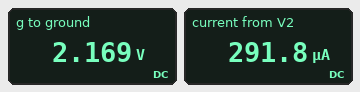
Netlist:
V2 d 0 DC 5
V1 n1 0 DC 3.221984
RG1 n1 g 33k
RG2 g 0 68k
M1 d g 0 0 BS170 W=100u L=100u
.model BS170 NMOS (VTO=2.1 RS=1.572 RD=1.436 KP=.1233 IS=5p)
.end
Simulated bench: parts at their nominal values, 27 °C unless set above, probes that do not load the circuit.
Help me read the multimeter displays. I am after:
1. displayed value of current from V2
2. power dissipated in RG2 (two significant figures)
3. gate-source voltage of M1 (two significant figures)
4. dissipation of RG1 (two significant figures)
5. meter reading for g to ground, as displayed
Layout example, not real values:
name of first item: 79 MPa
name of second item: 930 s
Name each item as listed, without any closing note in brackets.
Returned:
displayed value of current from V2: 291.8 µA
power dissipated in RG2: 69 µW
gate-source voltage of M1: 2.2 V
dissipation of RG1: 34 µW
meter reading for g to ground, as displayed: 2.169 V
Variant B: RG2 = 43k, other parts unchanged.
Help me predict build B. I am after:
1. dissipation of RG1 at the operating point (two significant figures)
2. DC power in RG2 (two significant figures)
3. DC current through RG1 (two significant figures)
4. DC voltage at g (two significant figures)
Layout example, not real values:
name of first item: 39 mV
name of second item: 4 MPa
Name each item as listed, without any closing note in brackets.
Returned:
dissipation of RG1 at the operating point: 59 µW
DC power in RG2: 77 µW
DC current through RG1: 42 µA
DC voltage at g: 1.8 V
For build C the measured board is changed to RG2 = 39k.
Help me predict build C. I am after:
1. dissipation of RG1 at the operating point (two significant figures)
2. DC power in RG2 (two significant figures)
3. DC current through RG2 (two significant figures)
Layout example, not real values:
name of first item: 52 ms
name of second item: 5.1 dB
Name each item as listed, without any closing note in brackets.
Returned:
dissipation of RG1 at the operating point: 66 µW
DC power in RG2: 78 µW
DC current through RG2: 45 µA
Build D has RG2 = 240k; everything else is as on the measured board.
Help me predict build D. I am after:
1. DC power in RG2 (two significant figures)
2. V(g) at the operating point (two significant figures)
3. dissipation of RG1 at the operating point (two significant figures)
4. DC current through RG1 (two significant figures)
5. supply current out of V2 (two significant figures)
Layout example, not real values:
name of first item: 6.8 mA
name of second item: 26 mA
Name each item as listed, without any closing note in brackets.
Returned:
DC power in RG2: 33 µW
V(g) at the operating point: 2.8 V
dissipation of RG1 at the operating point: 4.6 µW
DC current through RG1: 12 µA
supply current out of V2: 29 mA
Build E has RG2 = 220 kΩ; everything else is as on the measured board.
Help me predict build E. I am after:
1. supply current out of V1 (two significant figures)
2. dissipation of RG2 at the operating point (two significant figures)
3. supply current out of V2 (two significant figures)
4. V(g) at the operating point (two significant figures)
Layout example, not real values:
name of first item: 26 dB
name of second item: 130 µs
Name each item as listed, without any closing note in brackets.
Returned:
supply current out of V1: 13 µA
dissipation of RG2 at the operating point: 36 µW
supply current out of V2: 27 mA
V(g) at the operating point: 2.8 V
